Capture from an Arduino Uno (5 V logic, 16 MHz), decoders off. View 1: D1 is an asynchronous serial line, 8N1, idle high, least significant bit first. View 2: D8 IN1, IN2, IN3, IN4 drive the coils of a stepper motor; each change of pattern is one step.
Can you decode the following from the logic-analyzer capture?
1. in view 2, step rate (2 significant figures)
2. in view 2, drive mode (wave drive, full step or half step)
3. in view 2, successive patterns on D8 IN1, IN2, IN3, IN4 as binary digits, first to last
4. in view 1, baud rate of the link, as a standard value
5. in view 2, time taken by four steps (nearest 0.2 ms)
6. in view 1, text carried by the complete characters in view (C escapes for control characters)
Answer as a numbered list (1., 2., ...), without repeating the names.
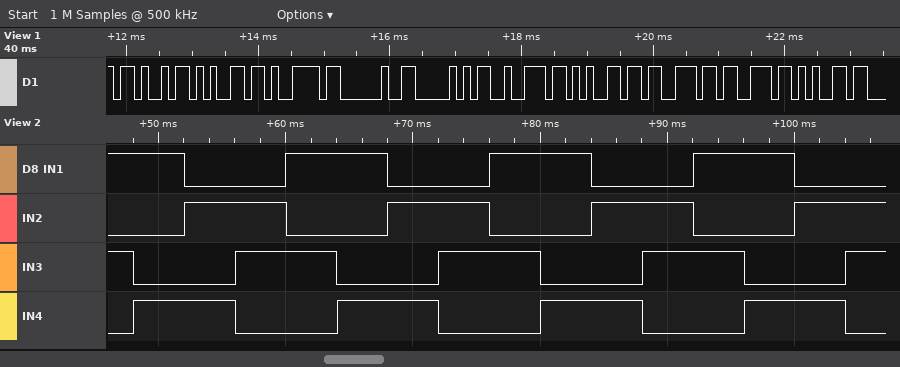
1. 250 steps/s
2. full step
3. 1010 1001 0101 0110 1010 1001 0101 0110 1010 1001 0101 0110 1010 1001 0101 0110
4. 9600 baud
5. 16.0 ms
6. "Key Presse"
